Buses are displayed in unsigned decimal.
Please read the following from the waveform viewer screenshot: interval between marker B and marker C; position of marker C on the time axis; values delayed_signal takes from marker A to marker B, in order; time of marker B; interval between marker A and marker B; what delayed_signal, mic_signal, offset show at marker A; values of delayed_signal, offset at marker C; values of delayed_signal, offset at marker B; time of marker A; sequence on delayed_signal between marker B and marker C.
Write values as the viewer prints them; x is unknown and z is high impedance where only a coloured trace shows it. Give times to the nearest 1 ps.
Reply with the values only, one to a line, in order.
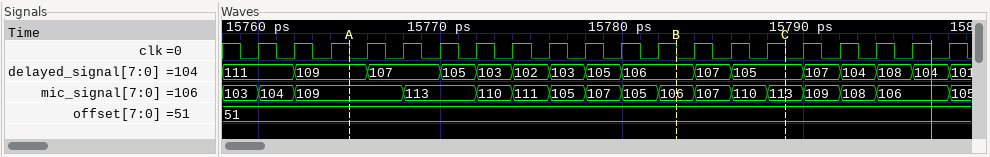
6 ps
15789 ps
109, 107, 105, 103, 102, 103, 105, 106
15783 ps
18 ps
delayed_signal=109, mic_signal=109, offset=51
delayed_signal=105, offset=51
delayed_signal=106, offset=51
15765 ps
106, 107, 105
